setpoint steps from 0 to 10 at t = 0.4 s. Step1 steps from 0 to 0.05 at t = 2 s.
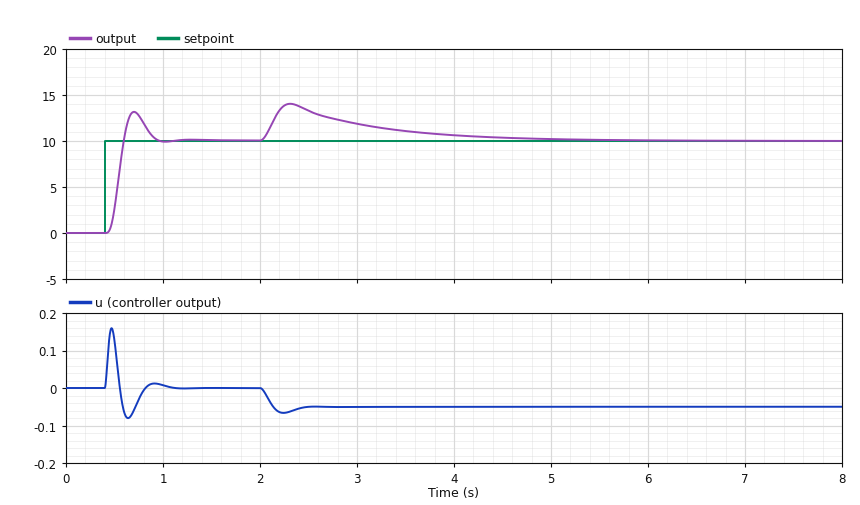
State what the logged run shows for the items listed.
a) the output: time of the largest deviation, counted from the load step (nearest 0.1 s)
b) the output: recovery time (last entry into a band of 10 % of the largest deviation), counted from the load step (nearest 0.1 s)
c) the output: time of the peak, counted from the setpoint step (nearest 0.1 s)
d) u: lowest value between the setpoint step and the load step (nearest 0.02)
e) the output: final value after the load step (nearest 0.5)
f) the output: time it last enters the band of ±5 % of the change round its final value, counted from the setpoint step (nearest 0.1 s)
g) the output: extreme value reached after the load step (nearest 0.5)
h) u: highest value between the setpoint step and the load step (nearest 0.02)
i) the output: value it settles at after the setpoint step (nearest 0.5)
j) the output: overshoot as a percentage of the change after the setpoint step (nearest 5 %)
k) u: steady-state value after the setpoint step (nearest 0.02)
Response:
0.3 s
2.4 s
0.3 s
-0.08
10.0
0.5 s
14.0
0.16
10.0
30 %
0.00
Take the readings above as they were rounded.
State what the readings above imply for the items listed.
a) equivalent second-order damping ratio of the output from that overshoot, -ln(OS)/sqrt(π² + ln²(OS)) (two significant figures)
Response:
0.36
